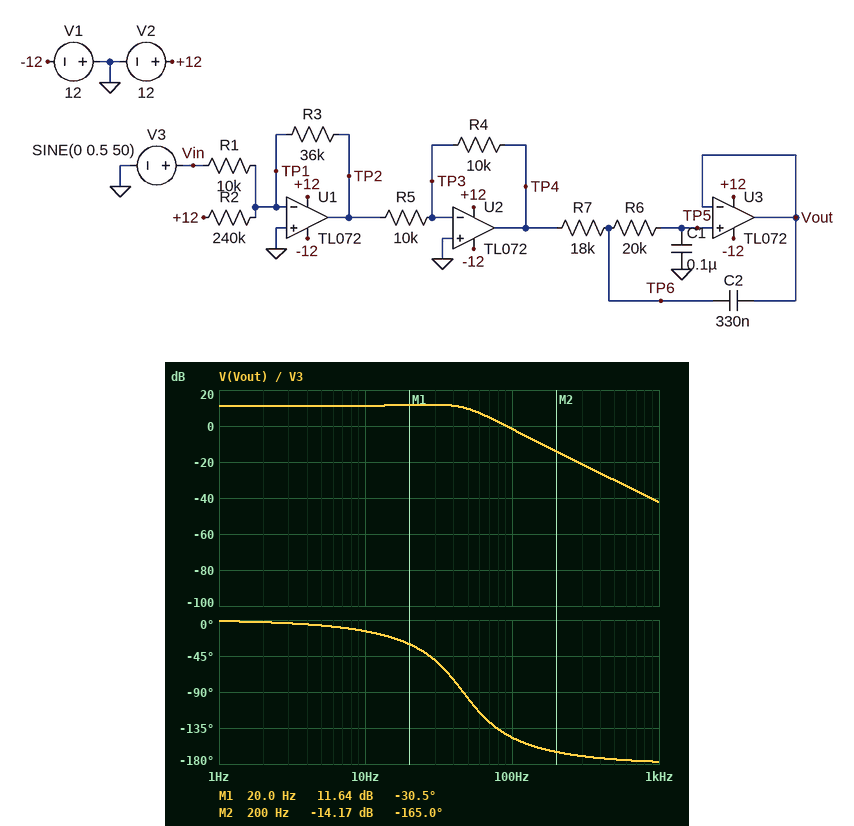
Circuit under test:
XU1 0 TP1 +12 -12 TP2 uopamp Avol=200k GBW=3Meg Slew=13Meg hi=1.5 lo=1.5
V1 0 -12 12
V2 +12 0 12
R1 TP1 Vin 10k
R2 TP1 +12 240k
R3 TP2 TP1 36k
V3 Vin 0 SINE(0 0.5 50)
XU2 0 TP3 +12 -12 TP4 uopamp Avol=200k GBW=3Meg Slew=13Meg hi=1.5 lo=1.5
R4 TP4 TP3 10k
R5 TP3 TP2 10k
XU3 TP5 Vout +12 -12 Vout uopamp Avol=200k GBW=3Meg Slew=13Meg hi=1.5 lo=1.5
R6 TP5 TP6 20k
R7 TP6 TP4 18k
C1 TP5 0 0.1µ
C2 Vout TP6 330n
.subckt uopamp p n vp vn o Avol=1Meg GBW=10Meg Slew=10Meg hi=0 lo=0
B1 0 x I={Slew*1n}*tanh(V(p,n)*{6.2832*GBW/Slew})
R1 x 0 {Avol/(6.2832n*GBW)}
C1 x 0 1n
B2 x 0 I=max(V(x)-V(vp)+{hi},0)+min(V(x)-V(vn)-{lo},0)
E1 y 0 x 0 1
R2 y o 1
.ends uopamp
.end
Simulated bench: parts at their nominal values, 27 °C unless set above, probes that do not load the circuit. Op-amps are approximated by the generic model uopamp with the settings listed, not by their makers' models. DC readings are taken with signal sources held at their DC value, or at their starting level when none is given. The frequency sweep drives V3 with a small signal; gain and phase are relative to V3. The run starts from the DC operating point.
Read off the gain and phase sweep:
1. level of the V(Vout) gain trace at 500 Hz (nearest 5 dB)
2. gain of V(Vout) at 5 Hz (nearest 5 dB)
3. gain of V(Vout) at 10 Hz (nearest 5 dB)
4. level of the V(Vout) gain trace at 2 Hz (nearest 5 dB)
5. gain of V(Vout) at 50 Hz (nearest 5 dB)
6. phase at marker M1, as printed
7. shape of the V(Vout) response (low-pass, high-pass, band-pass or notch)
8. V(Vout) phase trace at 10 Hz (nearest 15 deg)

-30 dB
10 dB
10 dB
10 dB
10 dB
-30.5 deg
low-pass
-15 deg
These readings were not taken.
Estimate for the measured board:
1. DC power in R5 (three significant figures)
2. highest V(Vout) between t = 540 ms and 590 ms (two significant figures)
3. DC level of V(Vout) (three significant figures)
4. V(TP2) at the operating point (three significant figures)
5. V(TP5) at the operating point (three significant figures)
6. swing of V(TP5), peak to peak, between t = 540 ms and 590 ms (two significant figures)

324 µW
3.3 V
1.80 V
-1.80 V
1.80 V
3.0 V
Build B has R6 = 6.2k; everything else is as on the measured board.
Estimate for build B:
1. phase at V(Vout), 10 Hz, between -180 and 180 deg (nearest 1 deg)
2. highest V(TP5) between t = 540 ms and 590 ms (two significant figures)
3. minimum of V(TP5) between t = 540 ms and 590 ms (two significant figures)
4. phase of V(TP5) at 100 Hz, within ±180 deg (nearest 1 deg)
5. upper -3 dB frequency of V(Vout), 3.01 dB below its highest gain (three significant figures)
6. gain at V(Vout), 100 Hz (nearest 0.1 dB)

-9 deg
3.6 V
-15 mV
-107 deg
90.2 Hz
7.1 dB
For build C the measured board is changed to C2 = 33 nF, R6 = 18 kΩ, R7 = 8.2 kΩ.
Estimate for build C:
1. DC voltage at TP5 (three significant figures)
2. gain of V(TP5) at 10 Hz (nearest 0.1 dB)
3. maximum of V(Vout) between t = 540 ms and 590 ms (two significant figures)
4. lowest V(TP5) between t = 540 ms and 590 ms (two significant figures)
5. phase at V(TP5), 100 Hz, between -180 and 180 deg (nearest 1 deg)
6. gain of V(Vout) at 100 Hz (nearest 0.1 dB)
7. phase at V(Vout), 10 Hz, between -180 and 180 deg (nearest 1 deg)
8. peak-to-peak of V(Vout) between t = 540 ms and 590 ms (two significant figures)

1.80 V
11.0 dB
3.2 V
370 mV
-64 deg
5.9 dB
-9 deg
2.9 V
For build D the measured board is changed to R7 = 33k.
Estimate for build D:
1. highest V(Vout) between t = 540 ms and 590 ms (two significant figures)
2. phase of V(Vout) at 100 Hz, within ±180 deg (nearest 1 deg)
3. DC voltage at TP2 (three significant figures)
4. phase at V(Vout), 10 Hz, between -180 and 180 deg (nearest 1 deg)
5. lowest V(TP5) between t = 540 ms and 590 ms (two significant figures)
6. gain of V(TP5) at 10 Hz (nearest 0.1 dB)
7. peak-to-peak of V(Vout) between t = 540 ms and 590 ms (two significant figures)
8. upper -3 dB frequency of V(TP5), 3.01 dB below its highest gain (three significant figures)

2.7 V
-156 deg
-1.80 V
-20 deg
910 mV
11.4 dB
1.8 V
38.7 Hz
